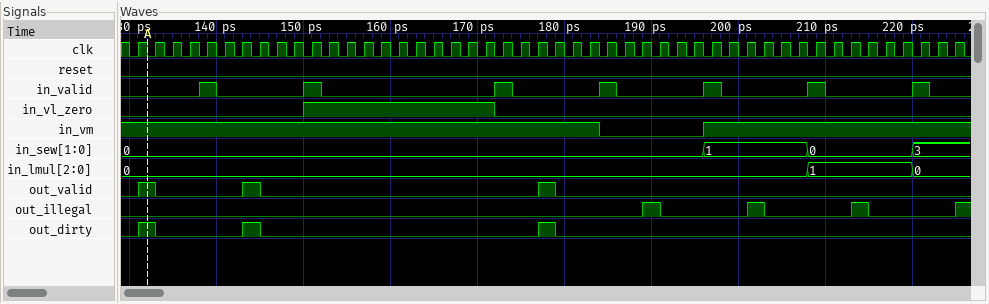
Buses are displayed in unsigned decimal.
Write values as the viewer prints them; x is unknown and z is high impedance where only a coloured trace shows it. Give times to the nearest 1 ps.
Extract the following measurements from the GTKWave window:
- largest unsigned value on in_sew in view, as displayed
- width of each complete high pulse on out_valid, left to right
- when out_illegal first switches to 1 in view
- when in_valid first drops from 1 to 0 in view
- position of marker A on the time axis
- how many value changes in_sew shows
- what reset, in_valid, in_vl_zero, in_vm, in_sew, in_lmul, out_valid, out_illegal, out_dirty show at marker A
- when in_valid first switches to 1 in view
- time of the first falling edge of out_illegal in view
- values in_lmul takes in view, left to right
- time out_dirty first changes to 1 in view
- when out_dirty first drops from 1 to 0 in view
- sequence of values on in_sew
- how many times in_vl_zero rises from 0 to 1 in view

3
2 ps, 2 ps, 2 ps
189 ps
140 ps
132 ps
3
reset=0, in_valid=0, in_vl_zero=0, in_vm=1, in_sew=0, in_lmul=0, out_valid=1, out_illegal=0, out_dirty=1
138 ps
191 ps
0, 1, 0
131 ps
133 ps
0, 1, 0, 3
1
